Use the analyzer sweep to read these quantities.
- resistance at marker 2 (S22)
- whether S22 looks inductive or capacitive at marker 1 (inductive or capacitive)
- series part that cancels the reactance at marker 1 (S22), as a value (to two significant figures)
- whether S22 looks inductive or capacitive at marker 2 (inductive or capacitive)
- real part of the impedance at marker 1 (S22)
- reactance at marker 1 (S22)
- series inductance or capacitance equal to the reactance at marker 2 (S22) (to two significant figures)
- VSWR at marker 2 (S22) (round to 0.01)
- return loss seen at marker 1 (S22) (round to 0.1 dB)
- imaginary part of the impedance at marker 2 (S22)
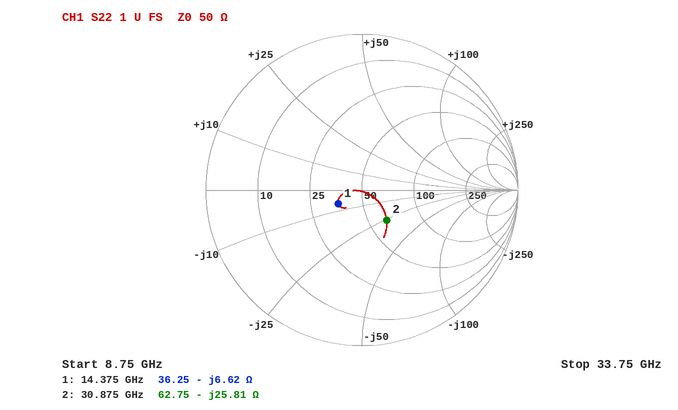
62.75 Ω
capacitive
73 pH
capacitive
36.25 Ω
-6.62 Ω
200 fF
1.66
15.1 dB
-25.81 Ω
